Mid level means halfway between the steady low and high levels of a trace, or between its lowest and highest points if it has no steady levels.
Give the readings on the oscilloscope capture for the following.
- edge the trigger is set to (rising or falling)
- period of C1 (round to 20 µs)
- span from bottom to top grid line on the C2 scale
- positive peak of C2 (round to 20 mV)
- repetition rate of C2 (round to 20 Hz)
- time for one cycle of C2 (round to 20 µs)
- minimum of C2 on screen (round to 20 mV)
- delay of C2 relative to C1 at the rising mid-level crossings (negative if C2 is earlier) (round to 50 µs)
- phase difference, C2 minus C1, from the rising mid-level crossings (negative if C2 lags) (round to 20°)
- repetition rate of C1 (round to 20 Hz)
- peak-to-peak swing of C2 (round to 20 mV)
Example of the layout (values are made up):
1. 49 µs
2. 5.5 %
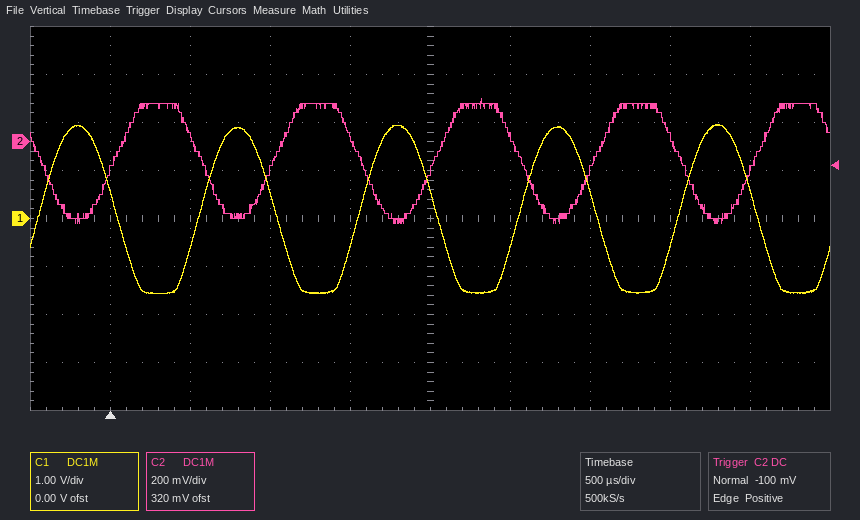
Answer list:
1. rising
2. 1.00 ms
3. 1.6 V
4. 180 mV
5. 1.00 kHz
6. 1.00 ms
7. -340 mV
8. +450 µs
9. -160°
10. 1.00 kHz
11. 520 mV
